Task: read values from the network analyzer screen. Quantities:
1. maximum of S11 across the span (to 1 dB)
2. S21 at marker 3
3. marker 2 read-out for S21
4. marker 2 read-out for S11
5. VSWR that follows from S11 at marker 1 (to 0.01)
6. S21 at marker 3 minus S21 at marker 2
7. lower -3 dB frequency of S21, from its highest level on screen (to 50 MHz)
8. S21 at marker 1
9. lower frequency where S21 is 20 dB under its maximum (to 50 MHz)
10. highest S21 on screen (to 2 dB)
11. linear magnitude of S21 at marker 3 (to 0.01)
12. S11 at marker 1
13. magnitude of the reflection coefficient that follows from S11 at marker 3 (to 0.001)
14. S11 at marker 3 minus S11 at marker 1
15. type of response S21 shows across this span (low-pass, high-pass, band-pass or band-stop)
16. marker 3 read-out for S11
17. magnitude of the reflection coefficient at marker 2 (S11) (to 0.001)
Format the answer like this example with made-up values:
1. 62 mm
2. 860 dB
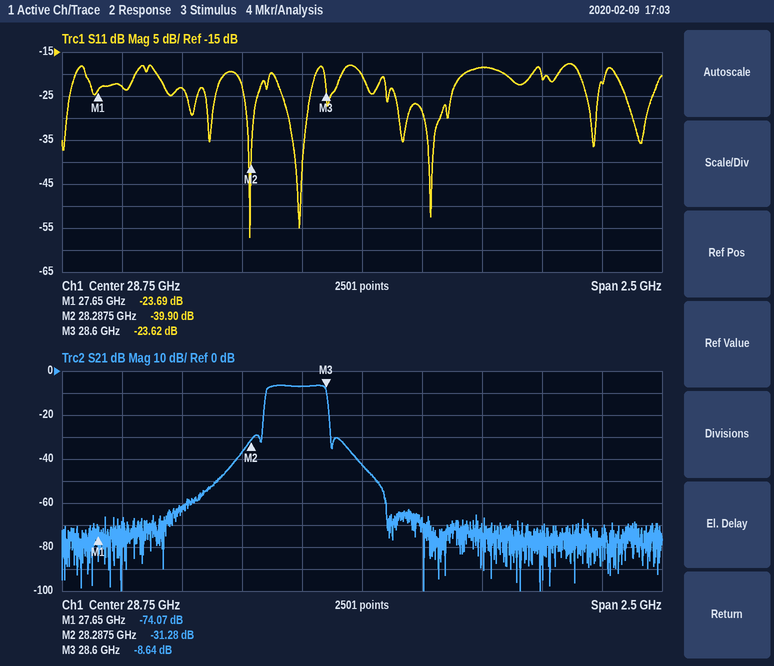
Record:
1. -18 dB
2. -8.64 dB
3. -31.28 dB
4. -39.90 dB
5. 1.14
6. 22.64 dB
7. 28.35 GHz
8. -74.07 dB
9. 28.35 GHz
10. -6 dB
11. 0.37
12. -23.69 dB
13. 0.066
14. 0.07 dB
15. band-pass
16. -23.62 dB
17. 0.010
